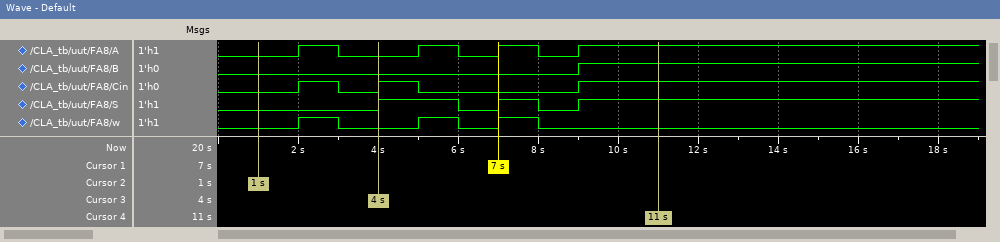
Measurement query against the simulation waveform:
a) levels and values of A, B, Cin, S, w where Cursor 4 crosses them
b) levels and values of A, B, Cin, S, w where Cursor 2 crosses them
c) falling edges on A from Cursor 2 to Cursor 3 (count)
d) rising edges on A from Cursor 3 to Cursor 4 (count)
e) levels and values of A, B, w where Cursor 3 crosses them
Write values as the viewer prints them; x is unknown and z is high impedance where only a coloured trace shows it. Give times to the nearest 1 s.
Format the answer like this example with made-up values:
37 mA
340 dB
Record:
A=1, B=1, Cin=1, S=1, w=0
A=0, B=0, Cin=0, S=0, w=0
1
3
A=0, B=0, w=0
